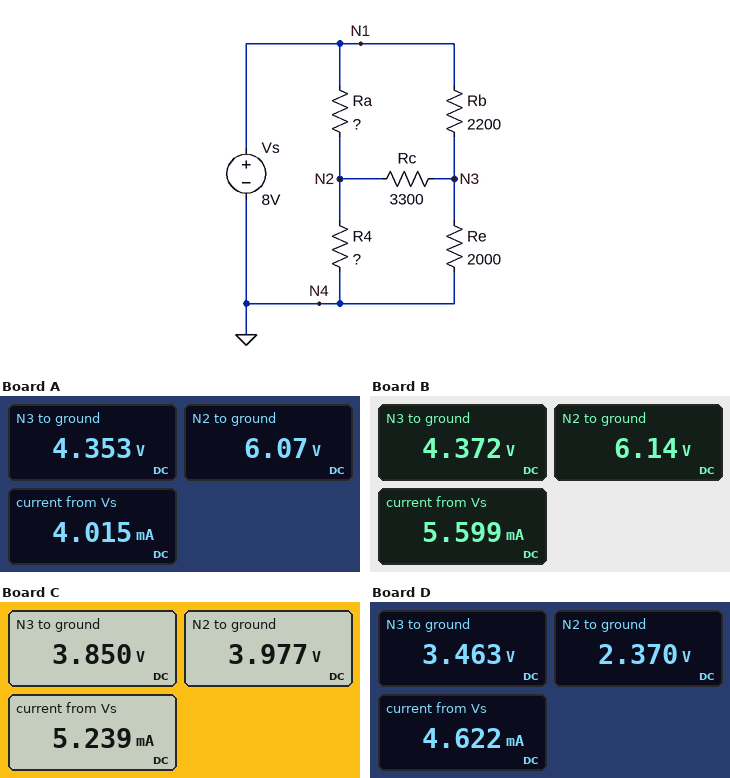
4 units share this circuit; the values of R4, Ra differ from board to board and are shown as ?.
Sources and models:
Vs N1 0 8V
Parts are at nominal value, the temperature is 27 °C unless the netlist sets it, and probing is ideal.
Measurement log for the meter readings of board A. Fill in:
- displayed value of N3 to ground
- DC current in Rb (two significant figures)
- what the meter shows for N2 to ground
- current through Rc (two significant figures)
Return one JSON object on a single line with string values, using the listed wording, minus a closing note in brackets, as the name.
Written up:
{"displayed value of N3 to ground": "4.353 V", "DC current in Rb": "1.7 mA", "what the meter shows for N2 to ground": "6.07 V", "current through Rc": "520 µA"}
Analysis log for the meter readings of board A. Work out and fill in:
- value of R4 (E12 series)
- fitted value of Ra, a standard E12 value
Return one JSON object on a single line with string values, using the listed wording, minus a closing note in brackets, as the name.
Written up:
{"value of R4": "3.3 kΩ", "fitted value of Ra, a standard E12 value": "820 Ω"}
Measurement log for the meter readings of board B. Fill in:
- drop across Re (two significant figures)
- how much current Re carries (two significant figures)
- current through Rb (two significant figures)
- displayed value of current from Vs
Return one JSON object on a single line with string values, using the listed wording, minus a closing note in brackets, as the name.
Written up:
{"drop across Re": "4.4 V", "how much current Re carries": "2.2 mA", "current through Rb": "1.6 mA", "displayed value of current from Vs": "5.599 mA"}
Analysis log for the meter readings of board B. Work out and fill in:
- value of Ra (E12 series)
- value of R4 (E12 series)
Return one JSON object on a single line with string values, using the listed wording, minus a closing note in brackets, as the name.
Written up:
{"value of Ra": "470 Ω", "value of R4": "1.8 kΩ"}
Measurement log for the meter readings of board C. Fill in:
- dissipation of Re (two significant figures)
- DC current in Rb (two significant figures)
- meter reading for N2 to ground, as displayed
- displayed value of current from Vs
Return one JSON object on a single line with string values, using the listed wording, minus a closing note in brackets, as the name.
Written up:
{"dissipation of Re": "7.4 mW", "DC current in Rb": "1.9 mA", "meter reading for N2 to ground, as displayed": "3.977 V", "displayed value of current from Vs": "5.239 mA"}
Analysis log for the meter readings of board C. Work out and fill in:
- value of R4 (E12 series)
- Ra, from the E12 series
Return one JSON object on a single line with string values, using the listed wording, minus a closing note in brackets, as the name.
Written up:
{"value of R4": "1.2 kΩ", "Ra, from the E12 series": "1.2 kΩ"}
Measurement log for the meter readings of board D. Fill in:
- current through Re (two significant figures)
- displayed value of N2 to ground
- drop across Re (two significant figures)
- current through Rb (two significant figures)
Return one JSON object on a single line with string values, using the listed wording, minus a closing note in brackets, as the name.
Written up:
{"current through Re": "1.7 mA", "displayed value of N2 to ground": "2.370 V", "drop across Re": "3.5 V", "current through Rb": "2.1 mA"}
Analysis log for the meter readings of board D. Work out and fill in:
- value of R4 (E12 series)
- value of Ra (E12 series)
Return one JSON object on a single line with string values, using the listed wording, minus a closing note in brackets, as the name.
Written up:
{"value of R4": "820 Ω", "value of Ra": "2.2 kΩ"}
